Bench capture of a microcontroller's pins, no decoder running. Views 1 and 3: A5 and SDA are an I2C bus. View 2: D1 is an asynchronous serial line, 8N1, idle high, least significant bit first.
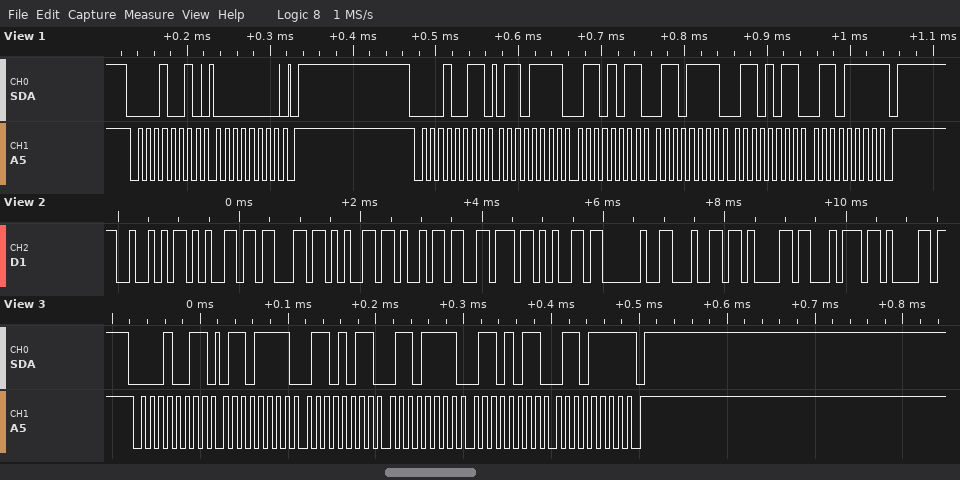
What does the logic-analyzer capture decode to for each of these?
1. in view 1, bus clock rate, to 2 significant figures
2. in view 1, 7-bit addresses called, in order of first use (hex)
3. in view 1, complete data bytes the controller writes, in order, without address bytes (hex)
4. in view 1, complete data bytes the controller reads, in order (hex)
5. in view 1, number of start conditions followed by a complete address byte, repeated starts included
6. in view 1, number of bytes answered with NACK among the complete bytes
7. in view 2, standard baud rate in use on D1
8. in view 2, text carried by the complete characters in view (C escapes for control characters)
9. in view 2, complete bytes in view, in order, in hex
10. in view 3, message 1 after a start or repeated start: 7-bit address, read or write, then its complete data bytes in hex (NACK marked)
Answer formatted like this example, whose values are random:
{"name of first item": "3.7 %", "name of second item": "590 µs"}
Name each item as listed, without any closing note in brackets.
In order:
{"in view 1, bus clock rate, to 2 significant figures": "100 kHz", "in view 1, 7-bit addresses called, in order of first use": "0x09", "in view 1, complete data bytes the controller writes, in order, without address bytes": "00", "in view 1, complete data bytes the controller reads, in order": "6F 6B 6F 6B 6F", "in view 1, number of start conditions followed by a complete address byte, repeated starts included": "2", "in view 1, number of bytes answered with NACK among the complete bytes": "1", "in view 2, standard baud rate in use on D1": "9600 baud", "in view 2, text carried by the complete characters in view": "\"Receive data\"", "in view 2, complete bytes in view, in order, in hex": "0x52 0x65 0x63 0x65 0x69 0x76 0x65 0x20 0x64 0x61 0x74 0x61", "in view 3, message 1 after a start or repeated start: 7-bit address, read or write, then its complete data bytes in hex": "0x09 read: 6F 6B 6F 6B 6F NACK"}
